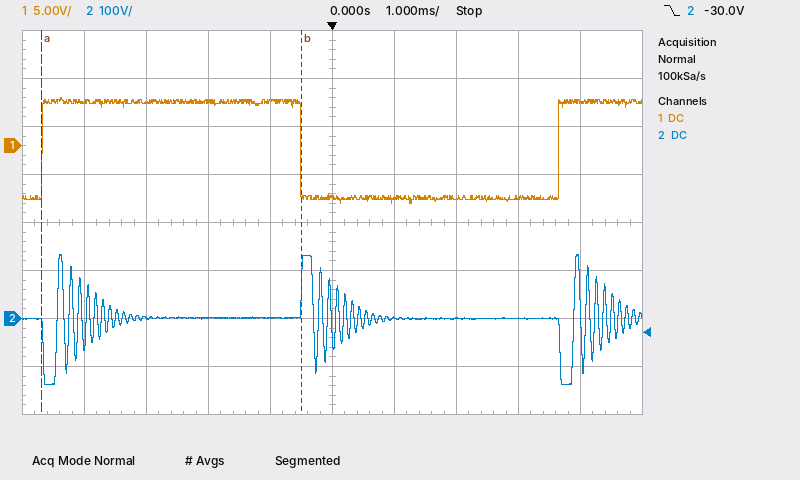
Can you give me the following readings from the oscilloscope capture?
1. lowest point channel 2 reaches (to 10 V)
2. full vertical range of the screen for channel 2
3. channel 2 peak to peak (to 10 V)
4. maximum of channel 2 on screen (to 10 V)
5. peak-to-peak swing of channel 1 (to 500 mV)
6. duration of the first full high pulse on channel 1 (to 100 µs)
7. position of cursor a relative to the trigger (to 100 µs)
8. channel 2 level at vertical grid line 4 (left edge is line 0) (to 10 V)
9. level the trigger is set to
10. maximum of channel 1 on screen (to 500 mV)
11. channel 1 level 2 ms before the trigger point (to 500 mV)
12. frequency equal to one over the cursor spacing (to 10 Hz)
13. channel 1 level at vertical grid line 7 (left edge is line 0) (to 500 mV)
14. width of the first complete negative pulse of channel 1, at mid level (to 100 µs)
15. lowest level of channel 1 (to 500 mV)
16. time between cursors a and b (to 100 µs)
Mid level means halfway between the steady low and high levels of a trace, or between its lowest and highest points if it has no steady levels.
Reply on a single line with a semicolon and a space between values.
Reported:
-140 V; 800 V; 270 V; 130 V; 11.0 V; 4.2 ms; -4.7 ms; 0 V; -30.0 V; 5.0 V; 4.5 V; 240 Hz; -5.5 V; 4.2 ms; -6.0 V; 4.2 ms
